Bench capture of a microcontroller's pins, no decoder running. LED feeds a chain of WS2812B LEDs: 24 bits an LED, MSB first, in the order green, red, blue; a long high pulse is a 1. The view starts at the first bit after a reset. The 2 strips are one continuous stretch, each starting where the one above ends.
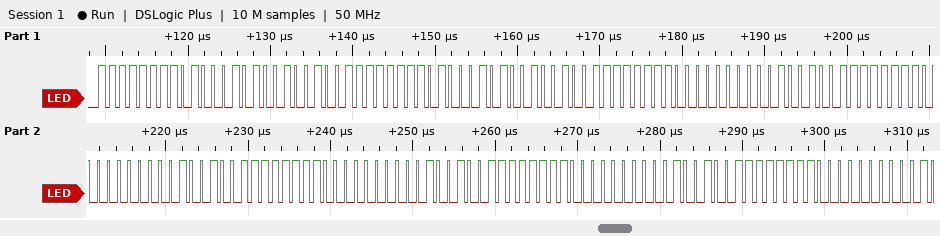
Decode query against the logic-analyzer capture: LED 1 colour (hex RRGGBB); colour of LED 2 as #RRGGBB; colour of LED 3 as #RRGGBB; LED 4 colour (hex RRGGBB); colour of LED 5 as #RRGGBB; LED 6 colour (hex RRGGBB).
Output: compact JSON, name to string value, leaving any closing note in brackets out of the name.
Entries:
{"LED 1 colour": "#45FF24", "colour of LED 2 as #RRGGBB": "#45FF24", "colour of LED 3 as #RRGGBB": "#00FF24", "LED 4 colour": "#00FF24", "colour of LED 5 as #RRGGBB": "#00FF24", "LED 6 colour": "#00FF24"}
